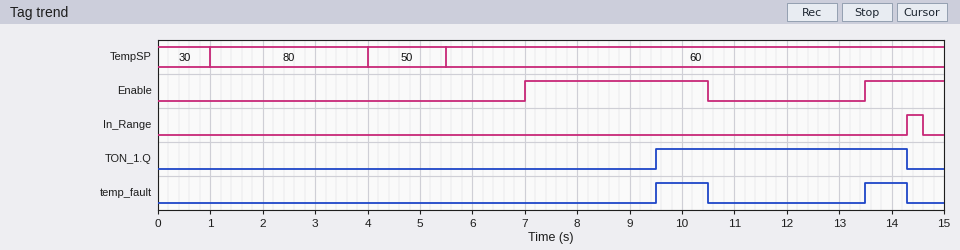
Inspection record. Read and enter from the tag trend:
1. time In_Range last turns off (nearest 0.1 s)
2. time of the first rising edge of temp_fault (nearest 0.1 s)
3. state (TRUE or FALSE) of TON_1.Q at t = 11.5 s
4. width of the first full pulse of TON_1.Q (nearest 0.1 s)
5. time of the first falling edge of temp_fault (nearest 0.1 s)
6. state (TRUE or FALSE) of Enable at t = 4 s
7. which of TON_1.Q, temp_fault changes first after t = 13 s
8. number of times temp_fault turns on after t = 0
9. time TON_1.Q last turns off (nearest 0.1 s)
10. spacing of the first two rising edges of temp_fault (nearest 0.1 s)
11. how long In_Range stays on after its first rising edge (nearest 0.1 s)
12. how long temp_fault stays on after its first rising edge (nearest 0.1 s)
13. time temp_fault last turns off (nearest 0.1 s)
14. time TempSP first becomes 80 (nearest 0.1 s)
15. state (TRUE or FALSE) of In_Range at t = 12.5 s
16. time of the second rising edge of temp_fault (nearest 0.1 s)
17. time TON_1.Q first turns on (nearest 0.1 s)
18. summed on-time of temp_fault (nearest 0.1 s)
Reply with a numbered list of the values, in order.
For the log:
1. 14.6 s
2. 9.5 s
3. TRUE
4. 4.8 s
5. 10.5 s
6. FALSE
7. temp_fault
8. 2
9. 14.3 s
10. 4.0 s
11. 0.3 s
12. 1.0 s
13. 14.3 s
14. 1.0 s
15. FALSE
16. 13.5 s
17. 9.5 s
18. 1.8 s
